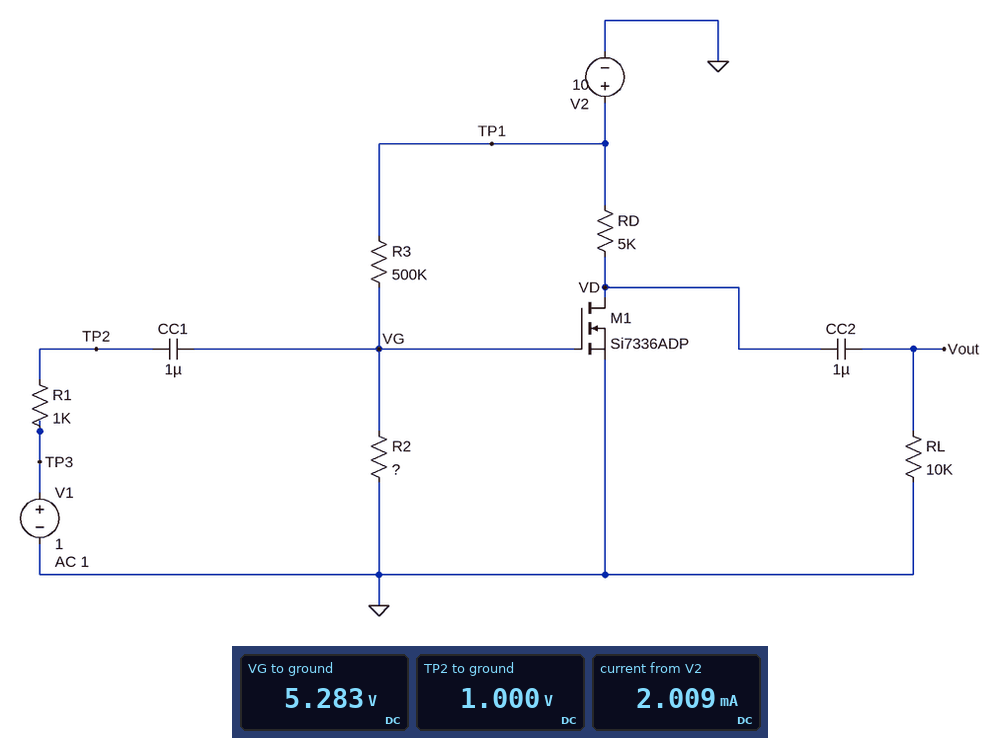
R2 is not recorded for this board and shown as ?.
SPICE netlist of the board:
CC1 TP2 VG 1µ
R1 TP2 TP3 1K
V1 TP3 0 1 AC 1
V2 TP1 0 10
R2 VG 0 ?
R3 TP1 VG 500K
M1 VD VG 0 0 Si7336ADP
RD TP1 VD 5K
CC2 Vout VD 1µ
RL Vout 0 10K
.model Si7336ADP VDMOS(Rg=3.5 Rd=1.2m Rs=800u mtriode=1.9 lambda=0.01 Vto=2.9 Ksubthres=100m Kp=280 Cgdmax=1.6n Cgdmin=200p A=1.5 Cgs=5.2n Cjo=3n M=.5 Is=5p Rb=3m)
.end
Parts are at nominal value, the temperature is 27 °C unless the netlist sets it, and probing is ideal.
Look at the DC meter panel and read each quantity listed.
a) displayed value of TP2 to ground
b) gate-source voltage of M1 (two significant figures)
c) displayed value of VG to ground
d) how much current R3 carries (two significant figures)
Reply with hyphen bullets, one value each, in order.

- 1.000 V
- 5.3 V
- 5.283 V
- 9.4 µA
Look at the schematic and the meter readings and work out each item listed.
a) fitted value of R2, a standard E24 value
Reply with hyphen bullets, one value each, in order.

- 560 kΩ
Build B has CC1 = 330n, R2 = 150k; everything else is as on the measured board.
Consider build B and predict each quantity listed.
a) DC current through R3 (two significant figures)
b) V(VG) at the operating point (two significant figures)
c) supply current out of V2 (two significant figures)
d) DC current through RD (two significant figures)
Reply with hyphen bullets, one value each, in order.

- 15 µA
- 2.3 V
- 26 µA
- 11 µA
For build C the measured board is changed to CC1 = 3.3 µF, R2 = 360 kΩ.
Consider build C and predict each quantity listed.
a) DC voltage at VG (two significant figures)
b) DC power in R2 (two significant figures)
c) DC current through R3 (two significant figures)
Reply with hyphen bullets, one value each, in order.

- 4.2 V
- 49 µW
- 12 µA
